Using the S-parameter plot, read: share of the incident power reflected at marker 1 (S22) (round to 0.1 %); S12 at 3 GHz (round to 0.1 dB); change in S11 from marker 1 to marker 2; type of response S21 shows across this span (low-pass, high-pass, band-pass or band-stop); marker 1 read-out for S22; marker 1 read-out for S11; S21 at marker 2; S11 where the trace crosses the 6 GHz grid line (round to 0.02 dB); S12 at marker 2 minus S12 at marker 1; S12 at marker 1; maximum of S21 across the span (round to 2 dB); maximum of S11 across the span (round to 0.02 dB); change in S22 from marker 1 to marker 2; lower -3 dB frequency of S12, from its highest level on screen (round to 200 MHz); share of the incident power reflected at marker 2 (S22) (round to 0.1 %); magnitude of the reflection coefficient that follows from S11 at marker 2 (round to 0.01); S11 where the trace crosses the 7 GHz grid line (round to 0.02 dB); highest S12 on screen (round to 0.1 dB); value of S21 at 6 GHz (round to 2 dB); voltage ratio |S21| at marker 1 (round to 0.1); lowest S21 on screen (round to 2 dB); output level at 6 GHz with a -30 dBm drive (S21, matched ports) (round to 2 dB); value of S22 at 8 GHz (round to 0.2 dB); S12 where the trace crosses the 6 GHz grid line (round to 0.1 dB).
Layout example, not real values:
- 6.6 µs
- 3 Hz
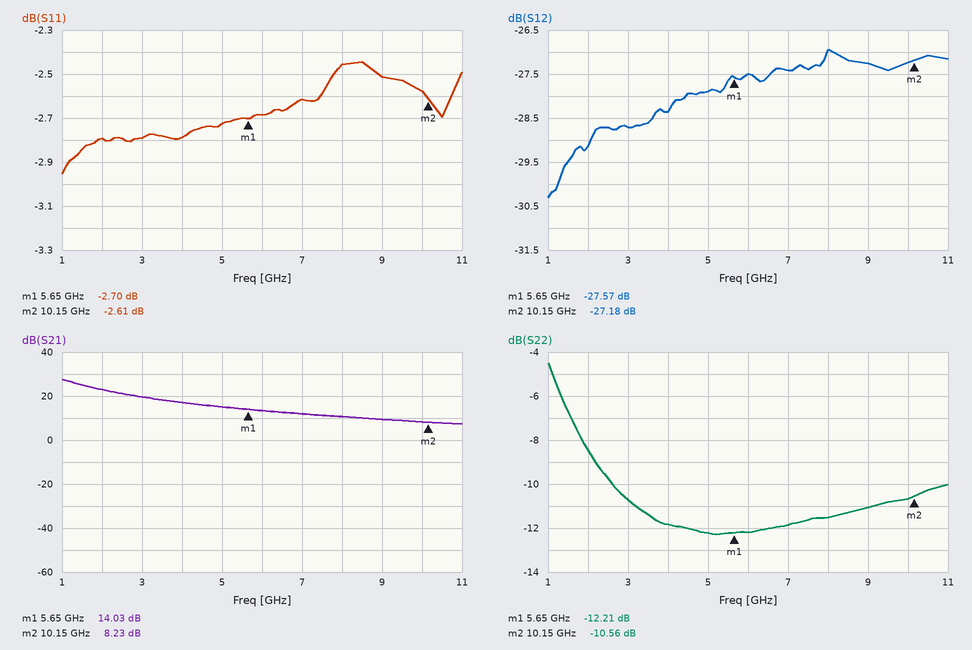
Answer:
- 6.0 %
- -28.7 dB
- 0.09 dB
- low-pass
- -12.21 dB
- -2.70 dB
- 8.23 dB
- -2.68 dB
- 0.39 dB
- -27.57 dB
- 28 dB
- -2.44 dB
- 1.65 dB
- 1.2 GHz
- 8.8 %
- 0.74
- -2.62 dB
- -26.9 dB
- 14 dB
- 5.0
- 8 dB
- -16 dBm
- -11.6 dB
- -27.5 dB
